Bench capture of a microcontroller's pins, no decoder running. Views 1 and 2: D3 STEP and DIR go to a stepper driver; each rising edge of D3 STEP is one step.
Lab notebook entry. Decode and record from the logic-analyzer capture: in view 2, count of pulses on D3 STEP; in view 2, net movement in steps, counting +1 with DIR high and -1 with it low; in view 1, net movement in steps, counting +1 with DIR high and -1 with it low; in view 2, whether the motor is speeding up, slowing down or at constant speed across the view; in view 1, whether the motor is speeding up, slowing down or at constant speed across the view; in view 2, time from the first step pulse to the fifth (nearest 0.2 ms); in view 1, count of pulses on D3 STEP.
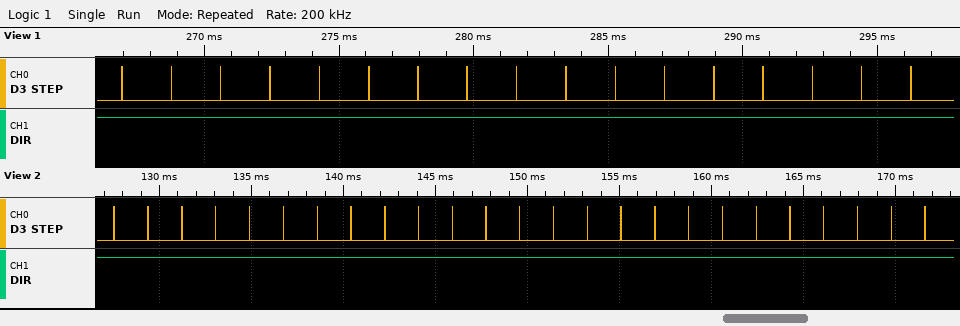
25
+25
+17
constant speed
constant speed
7.4 ms
17
